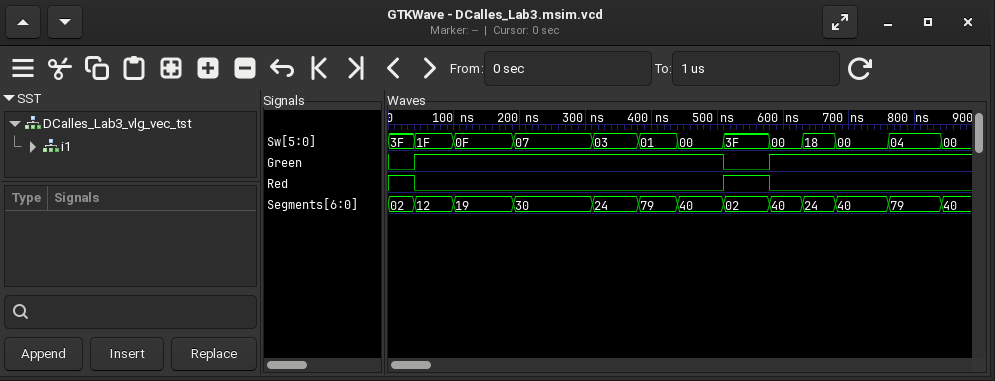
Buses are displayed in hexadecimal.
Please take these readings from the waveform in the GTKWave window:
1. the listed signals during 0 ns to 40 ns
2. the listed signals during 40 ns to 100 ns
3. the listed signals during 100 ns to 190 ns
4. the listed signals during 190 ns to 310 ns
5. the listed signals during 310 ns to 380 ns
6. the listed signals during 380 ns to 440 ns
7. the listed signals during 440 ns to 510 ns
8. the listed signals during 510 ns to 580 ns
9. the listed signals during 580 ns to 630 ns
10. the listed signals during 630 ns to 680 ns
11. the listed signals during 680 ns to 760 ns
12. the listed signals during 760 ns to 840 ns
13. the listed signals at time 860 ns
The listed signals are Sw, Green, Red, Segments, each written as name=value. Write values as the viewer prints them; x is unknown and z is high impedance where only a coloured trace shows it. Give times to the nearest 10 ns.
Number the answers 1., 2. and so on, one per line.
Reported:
1. Sw=3F, Green=0, Red=1, Segments=02
2. Sw=1F, Green=1, Red=0, Segments=12
3. Sw=0F, Green=1, Red=0, Segments=19
4. Sw=07, Green=1, Red=0, Segments=30
5. Sw=03, Green=1, Red=0, Segments=24
6. Sw=01, Green=1, Red=0, Segments=79
7. Sw=00, Green=1, Red=0, Segments=40
8. Sw=3F, Green=0, Red=1, Segments=02
9. Sw=00, Green=1, Red=0, Segments=40
10. Sw=18, Green=1, Red=0, Segments=24
11. Sw=00, Green=1, Red=0, Segments=40
12. Sw=04, Green=1, Red=0, Segments=79
13. Sw=00, Green=1, Red=0, Segments=40
